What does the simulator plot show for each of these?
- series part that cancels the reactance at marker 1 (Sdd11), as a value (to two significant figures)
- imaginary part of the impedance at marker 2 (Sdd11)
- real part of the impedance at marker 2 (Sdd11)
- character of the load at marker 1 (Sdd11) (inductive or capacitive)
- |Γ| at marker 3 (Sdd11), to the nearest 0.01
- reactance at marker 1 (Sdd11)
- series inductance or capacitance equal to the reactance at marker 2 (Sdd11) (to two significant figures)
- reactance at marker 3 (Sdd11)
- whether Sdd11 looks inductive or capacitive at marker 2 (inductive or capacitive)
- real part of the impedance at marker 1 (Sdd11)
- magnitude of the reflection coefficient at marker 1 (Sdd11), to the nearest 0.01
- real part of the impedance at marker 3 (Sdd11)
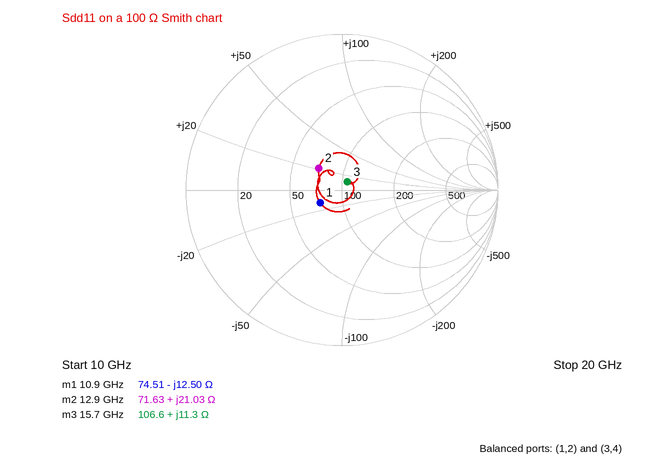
180 pH
+21.03 Ω
71.63 Ω
capacitive
0.06
-12.50 Ω
260 pH
+11.3 Ω
inductive
74.51 Ω
0.16
106.6 Ω
